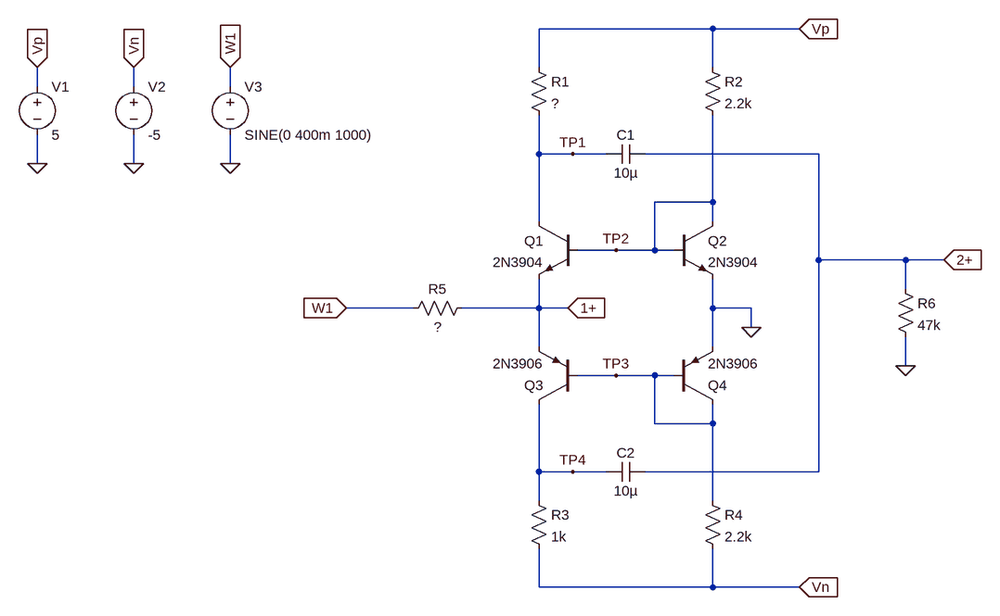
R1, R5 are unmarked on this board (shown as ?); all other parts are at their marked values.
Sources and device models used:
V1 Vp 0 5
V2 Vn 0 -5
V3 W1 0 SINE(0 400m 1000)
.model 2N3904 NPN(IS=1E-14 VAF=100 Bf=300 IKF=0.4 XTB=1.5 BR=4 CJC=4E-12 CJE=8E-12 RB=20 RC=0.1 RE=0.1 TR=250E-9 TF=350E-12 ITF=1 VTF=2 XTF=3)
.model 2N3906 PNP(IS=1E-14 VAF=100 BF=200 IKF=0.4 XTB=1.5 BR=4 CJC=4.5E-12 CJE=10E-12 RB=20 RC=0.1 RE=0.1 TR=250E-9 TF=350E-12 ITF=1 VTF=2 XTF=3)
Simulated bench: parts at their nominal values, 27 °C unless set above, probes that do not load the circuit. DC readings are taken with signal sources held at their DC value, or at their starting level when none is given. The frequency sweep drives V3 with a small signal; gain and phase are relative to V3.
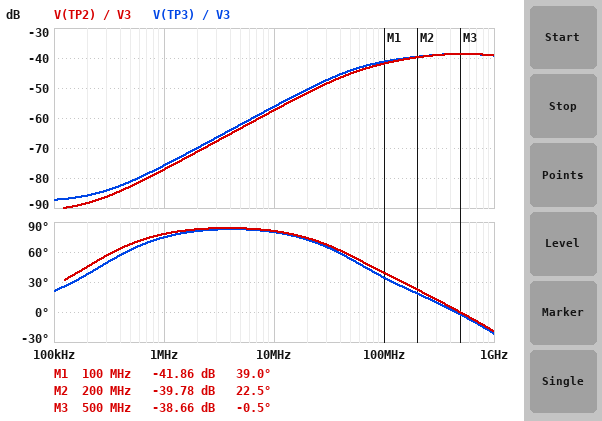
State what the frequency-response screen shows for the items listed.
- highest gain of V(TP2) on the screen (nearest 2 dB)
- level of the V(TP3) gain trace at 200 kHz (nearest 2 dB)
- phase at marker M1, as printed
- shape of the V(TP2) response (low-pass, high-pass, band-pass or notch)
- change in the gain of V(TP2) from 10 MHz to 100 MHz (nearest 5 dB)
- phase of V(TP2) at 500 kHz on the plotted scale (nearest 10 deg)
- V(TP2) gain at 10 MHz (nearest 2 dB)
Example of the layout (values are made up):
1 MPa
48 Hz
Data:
-38 dB
-86 dB
39.0 deg
high-pass
15 dB
70 deg
-58 dB
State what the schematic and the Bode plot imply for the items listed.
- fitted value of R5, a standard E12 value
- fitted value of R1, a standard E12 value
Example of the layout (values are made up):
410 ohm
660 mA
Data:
820 Ω
820 Ω
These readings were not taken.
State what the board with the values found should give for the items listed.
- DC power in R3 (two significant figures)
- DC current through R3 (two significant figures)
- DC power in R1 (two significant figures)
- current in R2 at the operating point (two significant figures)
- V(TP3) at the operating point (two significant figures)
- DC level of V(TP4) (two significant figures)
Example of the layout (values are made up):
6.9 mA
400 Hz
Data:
4.0 mW
2.0 mA
3.3 mW
2.0 mA
-670 mV
-3.0 V
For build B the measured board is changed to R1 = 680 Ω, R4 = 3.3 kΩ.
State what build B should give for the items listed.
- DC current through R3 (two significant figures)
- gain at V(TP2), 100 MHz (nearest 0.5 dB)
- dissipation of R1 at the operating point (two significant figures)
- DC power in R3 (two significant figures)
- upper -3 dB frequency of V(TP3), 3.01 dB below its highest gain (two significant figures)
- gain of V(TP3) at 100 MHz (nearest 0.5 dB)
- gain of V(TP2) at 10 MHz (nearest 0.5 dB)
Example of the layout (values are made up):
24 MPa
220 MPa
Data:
1.6 mA
-41.5 dB
1.8 mW
2.7 mW
2.0 GHz
-39.0 dB
-58.5 dB
